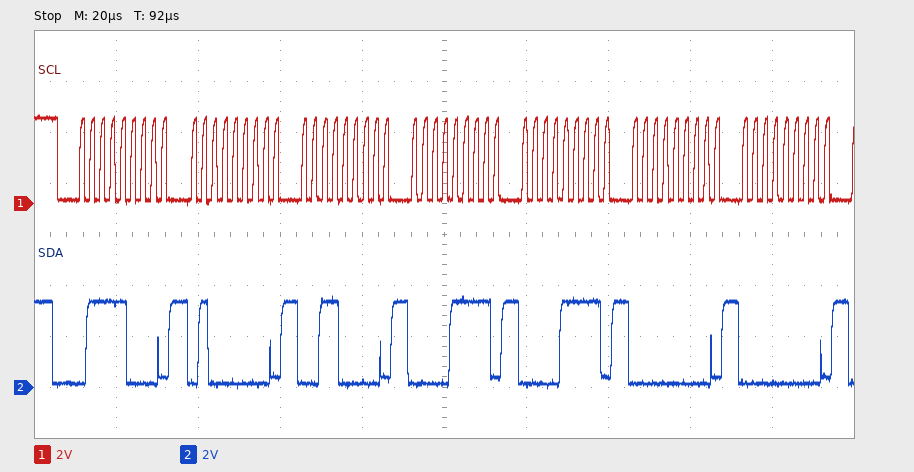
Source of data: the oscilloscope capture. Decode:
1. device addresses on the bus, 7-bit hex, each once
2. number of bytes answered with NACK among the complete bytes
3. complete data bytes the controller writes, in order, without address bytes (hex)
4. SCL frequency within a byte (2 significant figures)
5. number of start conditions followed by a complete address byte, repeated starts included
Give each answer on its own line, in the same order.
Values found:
0x3C
0
40 30 0F 0F 00 00
400 kHz
1
